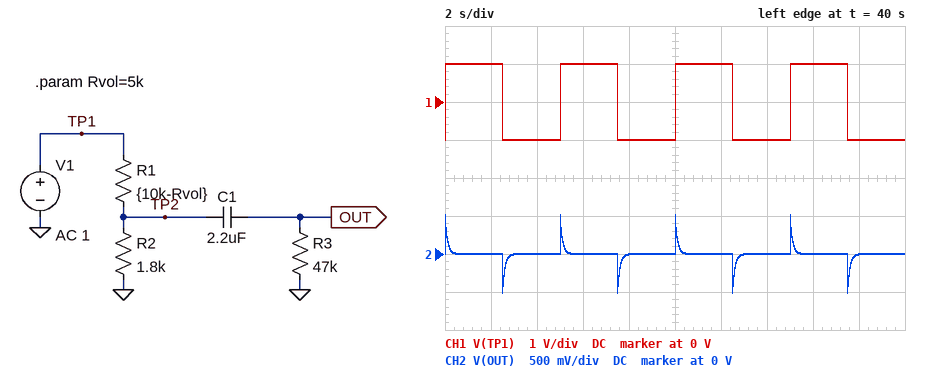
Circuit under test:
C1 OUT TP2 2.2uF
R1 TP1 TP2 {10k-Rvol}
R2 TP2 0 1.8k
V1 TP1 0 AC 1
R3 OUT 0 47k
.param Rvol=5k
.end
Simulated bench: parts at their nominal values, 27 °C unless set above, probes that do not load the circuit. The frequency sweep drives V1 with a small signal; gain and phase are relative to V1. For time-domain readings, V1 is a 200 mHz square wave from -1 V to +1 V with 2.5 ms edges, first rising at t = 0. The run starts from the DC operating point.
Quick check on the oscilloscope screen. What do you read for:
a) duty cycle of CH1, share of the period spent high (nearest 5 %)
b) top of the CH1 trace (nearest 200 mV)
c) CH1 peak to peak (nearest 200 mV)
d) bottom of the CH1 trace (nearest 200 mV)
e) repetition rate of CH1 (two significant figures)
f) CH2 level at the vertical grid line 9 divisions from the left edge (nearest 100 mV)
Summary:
50 %
1.0 V
2.0 V
-1.0 V
200 mHz
0 V
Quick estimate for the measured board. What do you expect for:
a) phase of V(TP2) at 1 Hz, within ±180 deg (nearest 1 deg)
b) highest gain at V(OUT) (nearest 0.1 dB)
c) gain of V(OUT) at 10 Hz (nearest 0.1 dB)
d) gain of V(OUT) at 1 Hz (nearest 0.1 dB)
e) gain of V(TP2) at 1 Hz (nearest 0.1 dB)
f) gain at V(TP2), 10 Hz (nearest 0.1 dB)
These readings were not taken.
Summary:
-1 deg
-11.8 dB
-11.9 dB
-16.9 dB
-11.6 dB
-11.8 dB
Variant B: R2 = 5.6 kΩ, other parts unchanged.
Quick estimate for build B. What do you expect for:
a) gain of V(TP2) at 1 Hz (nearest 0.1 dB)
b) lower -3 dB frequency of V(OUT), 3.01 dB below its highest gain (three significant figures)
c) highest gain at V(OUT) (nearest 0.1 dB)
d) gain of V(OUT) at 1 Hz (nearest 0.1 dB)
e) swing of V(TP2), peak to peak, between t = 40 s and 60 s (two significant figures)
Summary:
-5.7 dB
1.46 Hz
-6.0 dB
-11.0 dB
1.1 V
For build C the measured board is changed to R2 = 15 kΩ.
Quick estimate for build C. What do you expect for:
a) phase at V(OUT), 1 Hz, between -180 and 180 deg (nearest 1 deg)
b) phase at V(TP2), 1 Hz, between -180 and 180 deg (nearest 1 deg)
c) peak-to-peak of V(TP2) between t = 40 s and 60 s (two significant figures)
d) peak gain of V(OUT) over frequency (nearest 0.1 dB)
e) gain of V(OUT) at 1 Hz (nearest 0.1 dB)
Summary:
55 deg
-2 deg
1.5 V
-3.2 dB
-8.0 dB
